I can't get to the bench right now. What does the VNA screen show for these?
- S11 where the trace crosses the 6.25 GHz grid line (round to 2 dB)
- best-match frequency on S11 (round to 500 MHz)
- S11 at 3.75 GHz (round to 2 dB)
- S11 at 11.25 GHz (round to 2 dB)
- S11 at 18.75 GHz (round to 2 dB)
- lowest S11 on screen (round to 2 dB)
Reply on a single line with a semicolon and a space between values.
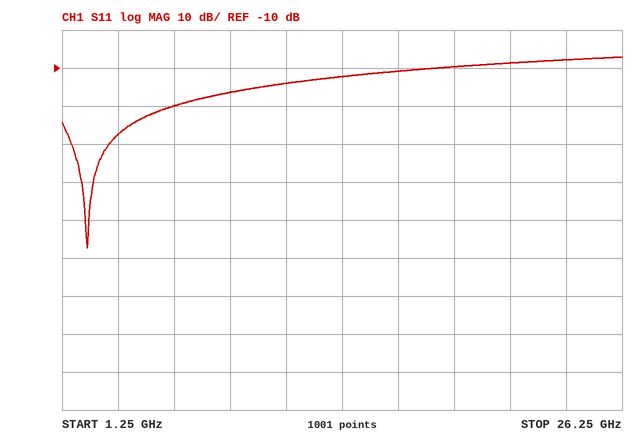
-20 dB; 2.5 GHz; -28 dB; -14 dB; -10 dB; -58 dB
